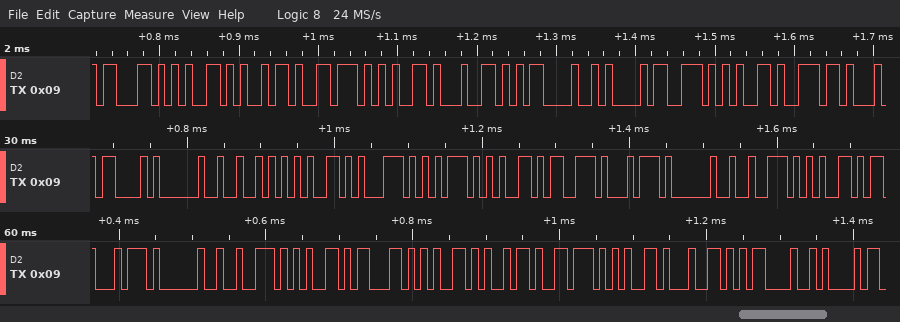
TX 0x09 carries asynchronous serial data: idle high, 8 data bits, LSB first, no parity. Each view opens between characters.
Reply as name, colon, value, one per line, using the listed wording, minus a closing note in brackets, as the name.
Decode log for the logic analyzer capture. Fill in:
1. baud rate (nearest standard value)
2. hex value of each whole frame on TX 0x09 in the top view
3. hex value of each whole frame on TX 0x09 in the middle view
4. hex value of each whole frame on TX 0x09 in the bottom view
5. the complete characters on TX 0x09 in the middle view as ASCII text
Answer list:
baud rate: 115200 baud
hex value of each whole frame on TX 0x09 in the top view: 63, 65, 69, 76, 65, 64, 0D, 0A, 73, 65, 6E
hex value of each whole frame on TX 0x09 in the middle view: 43, 20, 52, 65, 71, 75, 65, 73, 74, 20, 72, 65
hex value of each whole frame on TX 0x09 in the bottom view: 74, 20, 72, 65, 63, 65, 69, 76, 65, 64, 0D, 0A
the complete characters on TX 0x09 in the middle view as ASCII text: "C Request re"
